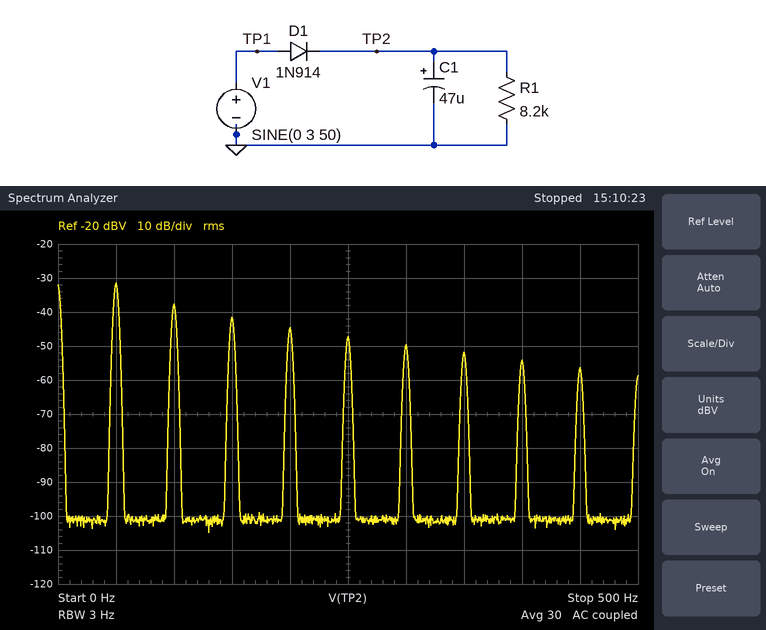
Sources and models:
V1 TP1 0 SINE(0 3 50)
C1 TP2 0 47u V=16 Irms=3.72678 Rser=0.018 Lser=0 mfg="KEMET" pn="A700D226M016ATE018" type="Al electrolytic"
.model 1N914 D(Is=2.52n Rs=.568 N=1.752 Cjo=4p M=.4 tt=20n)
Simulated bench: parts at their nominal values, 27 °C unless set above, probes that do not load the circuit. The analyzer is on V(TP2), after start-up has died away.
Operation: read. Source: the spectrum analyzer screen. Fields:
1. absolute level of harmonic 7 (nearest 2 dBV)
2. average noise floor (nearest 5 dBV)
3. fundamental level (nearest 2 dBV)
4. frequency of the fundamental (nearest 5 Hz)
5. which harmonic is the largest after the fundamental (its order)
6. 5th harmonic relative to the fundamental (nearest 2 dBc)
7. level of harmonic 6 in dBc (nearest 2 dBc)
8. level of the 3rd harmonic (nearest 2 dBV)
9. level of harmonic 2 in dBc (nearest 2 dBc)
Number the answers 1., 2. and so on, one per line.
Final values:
1. -52 dBV
2. -100 dBV
3. -32 dBV
4. 50 Hz
5. 2
6. -16 dBc
7. -18 dBc
8. -42 dBV
9. -6 dBc
